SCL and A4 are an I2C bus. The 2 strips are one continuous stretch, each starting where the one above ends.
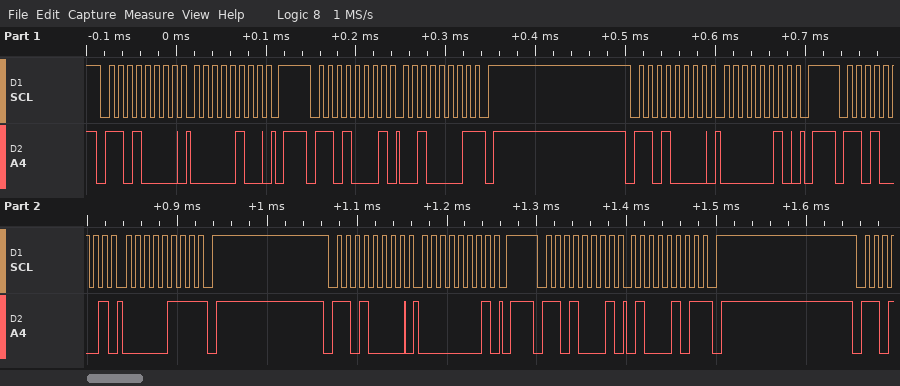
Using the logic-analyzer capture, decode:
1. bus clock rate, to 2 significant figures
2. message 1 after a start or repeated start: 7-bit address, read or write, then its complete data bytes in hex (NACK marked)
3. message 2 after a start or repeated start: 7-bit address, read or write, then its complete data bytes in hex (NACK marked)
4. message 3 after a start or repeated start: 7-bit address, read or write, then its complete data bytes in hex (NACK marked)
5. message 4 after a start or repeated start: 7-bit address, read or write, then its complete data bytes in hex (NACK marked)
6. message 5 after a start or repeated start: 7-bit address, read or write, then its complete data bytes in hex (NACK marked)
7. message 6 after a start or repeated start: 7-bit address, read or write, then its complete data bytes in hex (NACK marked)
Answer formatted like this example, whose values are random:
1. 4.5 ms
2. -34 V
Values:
1. 100 kHz
2. 0x68 write: 04
3. 0x68 read: 21 NACK
4. 0x68 write: 02
5. 0x68 read: 07 NACK
6. 0x68 write: 01
7. 0x68 read: 45 NACK
